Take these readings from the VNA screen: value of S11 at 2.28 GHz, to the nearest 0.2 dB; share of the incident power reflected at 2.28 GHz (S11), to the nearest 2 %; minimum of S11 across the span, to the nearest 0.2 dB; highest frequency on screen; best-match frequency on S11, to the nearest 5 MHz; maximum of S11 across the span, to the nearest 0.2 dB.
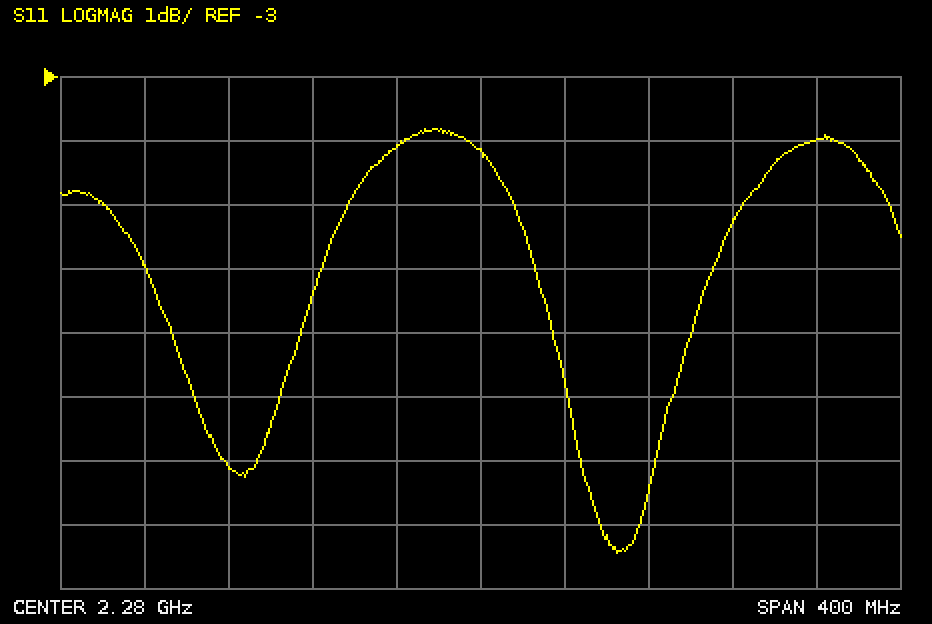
-4.2 dB
38 %
-10.4 dB
2.48 GHz
2.345 GHz
-3.8 dB
